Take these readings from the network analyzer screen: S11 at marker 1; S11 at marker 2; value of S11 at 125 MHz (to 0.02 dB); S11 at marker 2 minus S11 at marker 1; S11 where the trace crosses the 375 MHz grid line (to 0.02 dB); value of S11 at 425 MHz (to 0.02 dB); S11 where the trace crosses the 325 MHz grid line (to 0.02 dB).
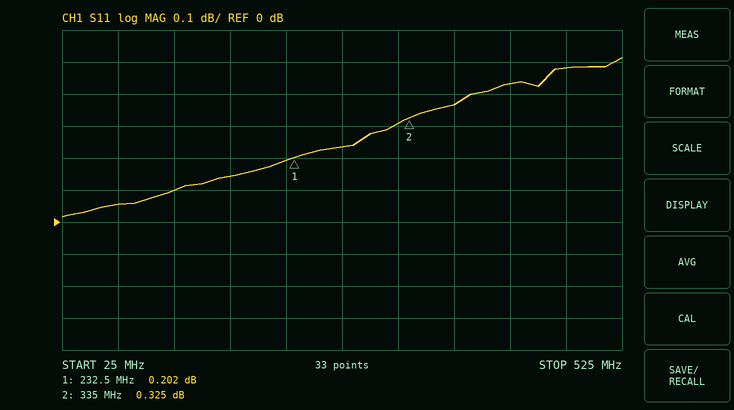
0.202 dB
0.325 dB
0.10 dB
0.123 dB
0.36 dB
0.44 dB
0.30 dB
